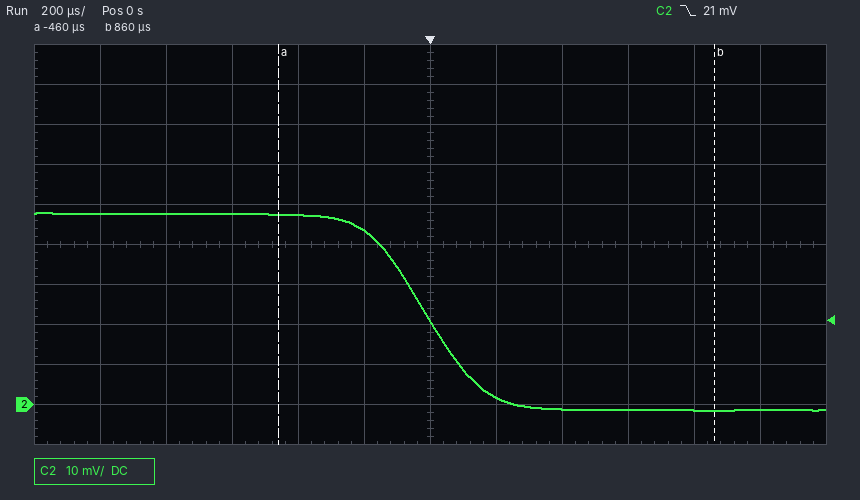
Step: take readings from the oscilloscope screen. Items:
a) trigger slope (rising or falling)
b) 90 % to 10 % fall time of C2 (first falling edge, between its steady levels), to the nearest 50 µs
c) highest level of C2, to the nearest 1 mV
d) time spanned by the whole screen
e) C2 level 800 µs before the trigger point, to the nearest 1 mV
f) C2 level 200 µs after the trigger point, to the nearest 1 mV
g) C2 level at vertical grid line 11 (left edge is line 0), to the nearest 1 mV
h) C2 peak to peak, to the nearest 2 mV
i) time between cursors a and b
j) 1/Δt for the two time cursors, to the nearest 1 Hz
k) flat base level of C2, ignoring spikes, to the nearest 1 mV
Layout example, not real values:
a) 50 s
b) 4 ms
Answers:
a) falling
b) 350 µs
c) 48 mV
d) 2.4 ms
e) 48 mV
f) 2 mV
g) -1 mV
h) 50 mV
i) 1.32 ms
j) 758 Hz
k) -1 mV
